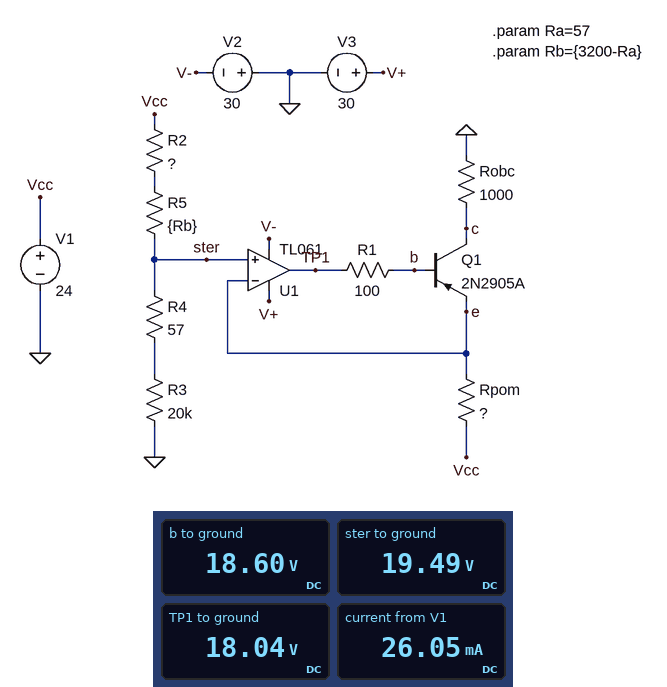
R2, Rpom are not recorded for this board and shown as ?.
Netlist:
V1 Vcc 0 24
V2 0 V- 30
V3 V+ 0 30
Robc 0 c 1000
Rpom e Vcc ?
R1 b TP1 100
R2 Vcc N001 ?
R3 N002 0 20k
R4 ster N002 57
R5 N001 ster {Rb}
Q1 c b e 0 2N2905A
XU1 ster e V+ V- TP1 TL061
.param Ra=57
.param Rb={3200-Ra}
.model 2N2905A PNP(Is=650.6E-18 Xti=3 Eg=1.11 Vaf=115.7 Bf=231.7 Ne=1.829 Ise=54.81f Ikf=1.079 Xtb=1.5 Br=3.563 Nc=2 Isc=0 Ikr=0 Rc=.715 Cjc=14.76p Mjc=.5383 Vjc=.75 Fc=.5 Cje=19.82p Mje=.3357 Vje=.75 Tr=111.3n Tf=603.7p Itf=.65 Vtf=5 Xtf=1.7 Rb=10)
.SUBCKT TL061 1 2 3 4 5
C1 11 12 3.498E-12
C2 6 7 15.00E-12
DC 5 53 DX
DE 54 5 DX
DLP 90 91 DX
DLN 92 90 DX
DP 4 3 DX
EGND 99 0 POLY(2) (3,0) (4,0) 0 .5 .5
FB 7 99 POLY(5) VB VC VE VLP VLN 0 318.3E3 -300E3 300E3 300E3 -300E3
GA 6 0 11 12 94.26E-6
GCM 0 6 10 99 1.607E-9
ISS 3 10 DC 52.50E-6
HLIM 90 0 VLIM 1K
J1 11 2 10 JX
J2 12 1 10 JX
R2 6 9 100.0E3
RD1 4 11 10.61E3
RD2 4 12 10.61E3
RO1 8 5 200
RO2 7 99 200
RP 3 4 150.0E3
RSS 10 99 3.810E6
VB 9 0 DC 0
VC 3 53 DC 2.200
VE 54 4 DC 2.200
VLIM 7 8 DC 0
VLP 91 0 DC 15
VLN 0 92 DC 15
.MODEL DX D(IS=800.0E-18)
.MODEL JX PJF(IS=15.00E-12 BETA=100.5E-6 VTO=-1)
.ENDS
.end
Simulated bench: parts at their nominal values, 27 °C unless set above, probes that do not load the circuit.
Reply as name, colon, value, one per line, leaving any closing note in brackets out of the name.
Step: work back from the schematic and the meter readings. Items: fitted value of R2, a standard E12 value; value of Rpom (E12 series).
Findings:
fitted value of R2, a standard E12 value: 1.5 kΩ
value of Rpom: 180 Ω
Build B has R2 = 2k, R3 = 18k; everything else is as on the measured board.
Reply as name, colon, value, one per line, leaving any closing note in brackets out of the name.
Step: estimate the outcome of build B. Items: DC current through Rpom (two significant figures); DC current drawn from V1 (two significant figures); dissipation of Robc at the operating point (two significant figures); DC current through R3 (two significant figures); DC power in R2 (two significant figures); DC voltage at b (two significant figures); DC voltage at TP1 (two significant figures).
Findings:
DC current through Rpom: 30 mA
DC current drawn from V1: 31 mA
dissipation of Robc at the operating point: 350 mW
DC current through R3: 1.0 mA
DC power in R2: 2.1 mW
DC voltage at b: 18 V
DC voltage at TP1: 17 V
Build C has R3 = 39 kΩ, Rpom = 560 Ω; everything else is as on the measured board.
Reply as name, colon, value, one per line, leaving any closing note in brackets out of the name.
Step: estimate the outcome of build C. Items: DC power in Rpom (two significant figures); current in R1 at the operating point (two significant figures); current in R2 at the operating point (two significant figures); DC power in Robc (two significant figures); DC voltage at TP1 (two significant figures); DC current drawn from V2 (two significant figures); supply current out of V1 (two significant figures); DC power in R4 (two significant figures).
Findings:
DC power in Rpom: 12 mW
current in R1 at the operating point: 18 µA
current in R2 at the operating point: 550 µA
DC power in Robc: 21 mW
DC voltage at TP1: 21 V
DC current drawn from V2: 450 µA
supply current out of V1: 5.1 mA
DC power in R4: 17 µW
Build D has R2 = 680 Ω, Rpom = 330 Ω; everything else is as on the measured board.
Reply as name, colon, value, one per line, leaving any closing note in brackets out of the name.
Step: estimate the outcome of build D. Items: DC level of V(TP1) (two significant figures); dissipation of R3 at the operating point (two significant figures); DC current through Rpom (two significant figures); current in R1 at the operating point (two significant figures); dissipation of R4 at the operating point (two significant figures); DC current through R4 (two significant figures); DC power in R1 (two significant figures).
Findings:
DC level of V(TP1): 19 V
dissipation of R3 at the operating point: 20 mW
DC current through Rpom: 12 mA
current in R1 at the operating point: 48 µA
dissipation of R4 at the operating point: 58 µW
DC current through R4: 1.0 mA
DC power in R1: 230 nW
